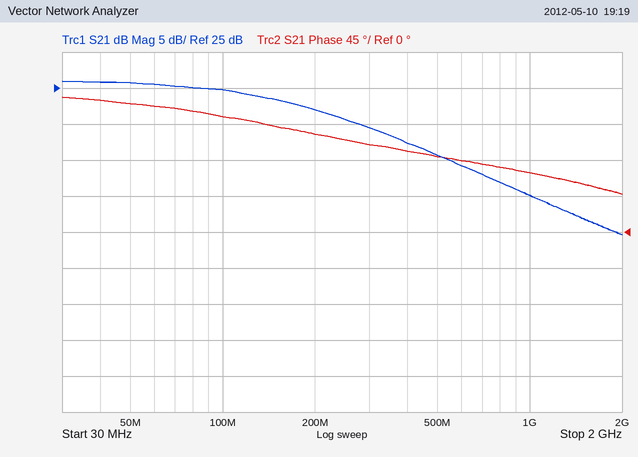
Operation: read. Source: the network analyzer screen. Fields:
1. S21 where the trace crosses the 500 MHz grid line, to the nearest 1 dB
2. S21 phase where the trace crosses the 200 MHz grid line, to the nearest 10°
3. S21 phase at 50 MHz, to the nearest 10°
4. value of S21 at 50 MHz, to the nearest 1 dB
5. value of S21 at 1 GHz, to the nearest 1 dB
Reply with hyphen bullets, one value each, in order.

- 16 dB
- 120°
- 160°
- 26 dB
- 10 dB
